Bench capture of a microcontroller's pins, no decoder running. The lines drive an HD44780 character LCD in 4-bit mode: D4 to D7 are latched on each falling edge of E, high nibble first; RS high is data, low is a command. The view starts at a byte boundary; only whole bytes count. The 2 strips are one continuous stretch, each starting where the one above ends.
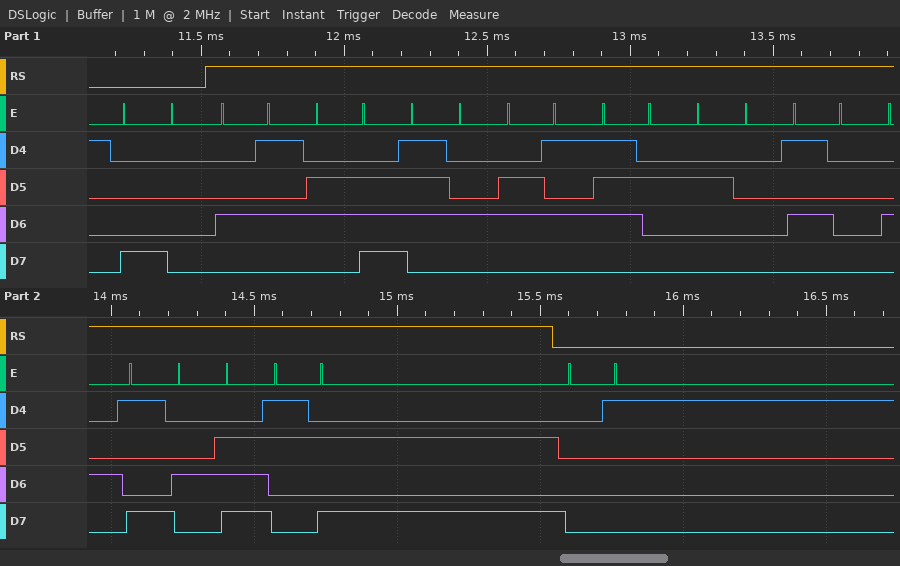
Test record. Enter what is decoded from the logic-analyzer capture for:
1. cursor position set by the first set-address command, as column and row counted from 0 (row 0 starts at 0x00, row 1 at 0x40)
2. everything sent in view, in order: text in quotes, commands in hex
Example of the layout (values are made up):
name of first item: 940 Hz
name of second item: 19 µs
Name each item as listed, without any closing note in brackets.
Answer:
cursor position set by the first set-address command, as column and row counted from 0: column 0, row 0
everything sent in view, in order: text in quotes, commands in hex: 0x80 "Enter PIN:" 0x01
